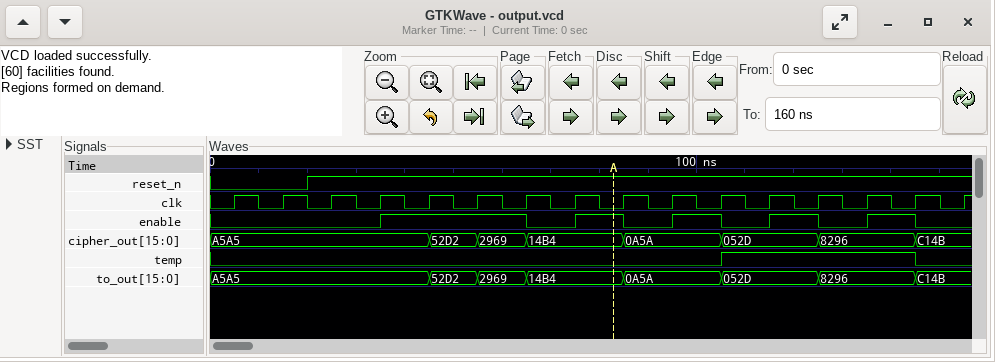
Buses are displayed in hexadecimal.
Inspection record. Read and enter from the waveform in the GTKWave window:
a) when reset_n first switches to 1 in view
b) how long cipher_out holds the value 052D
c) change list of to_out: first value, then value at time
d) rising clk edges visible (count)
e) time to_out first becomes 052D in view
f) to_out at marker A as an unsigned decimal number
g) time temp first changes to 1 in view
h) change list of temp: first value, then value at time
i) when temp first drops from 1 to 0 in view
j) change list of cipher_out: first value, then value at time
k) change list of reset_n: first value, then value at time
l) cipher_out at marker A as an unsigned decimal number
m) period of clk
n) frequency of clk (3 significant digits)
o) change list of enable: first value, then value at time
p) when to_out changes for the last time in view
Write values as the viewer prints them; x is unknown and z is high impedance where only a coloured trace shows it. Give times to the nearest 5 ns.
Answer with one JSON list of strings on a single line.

["20 ns", "20 ns", "A5A5, 52D2 at 45 ns, 2969 at 55 ns, 14B4 at 65 ns, 0A5A at 85 ns, 052D at 105 ns, 8296 at 125 ns, C14B at 145 ns", "16", "105 ns", "5300", "105 ns", "0, 1 at 105 ns, 0 at 145 ns", "145 ns", "A5A5, 52D2 at 45 ns, 2969 at 55 ns, 14B4 at 65 ns, 0A5A at 85 ns, 052D at 105 ns, 8296 at 125 ns, C14B at 145 ns", "0, 1 at 20 ns", "5300", "10 ns", "100 MHz", "0, 1 at 35 ns, 0 at 65 ns, 1 at 75 ns, 0 at 85 ns, 1 at 95 ns, 0 at 105 ns, 1 at 115 ns, 0 at 125 ns, 1 at 135 ns, 0 at 145 ns", "145 ns"]
